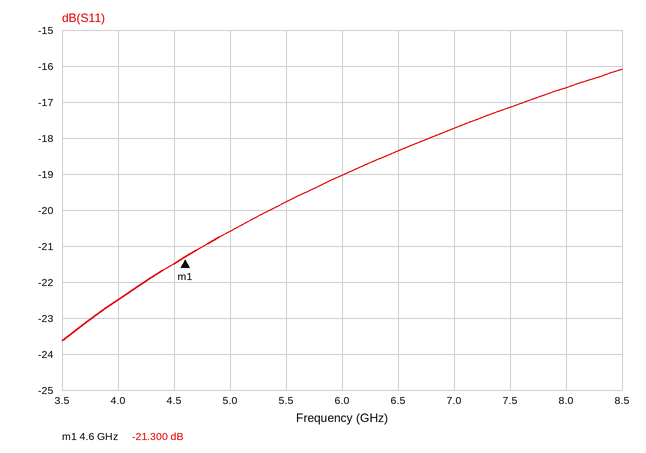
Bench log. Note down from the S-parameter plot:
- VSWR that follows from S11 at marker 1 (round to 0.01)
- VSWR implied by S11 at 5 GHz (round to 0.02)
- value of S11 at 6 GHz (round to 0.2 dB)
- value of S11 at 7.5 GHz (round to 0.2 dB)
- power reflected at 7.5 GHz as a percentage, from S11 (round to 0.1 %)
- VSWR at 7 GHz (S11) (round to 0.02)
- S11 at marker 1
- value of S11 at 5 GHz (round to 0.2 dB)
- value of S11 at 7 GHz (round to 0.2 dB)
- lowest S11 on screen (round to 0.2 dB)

1.19
1.20
-19.0 dB
-17.2 dB
1.9 %
1.30
-21.300 dB
-20.6 dB
-17.8 dB
-23.6 dB
